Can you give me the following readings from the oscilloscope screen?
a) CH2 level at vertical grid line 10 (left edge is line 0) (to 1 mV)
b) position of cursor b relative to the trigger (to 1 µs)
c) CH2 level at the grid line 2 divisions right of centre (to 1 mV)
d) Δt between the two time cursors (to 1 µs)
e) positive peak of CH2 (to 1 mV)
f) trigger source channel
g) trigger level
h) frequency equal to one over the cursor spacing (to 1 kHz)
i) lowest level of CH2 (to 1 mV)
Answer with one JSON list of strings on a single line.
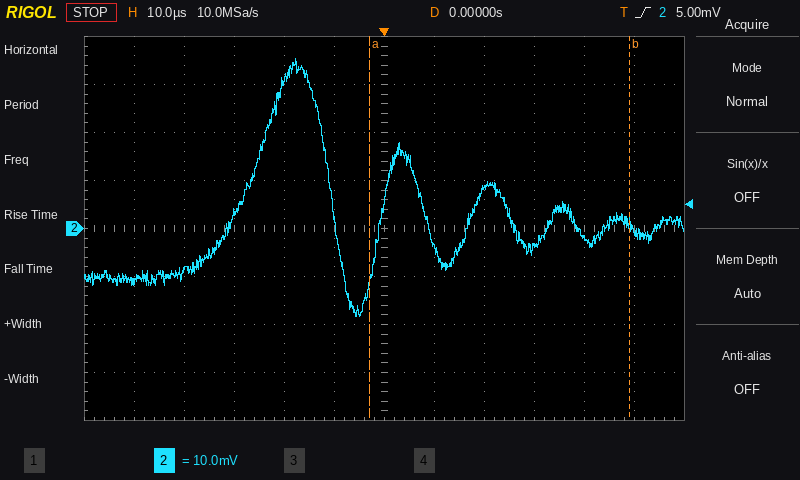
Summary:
["-2 mV", "+49 µs", "8 mV", "52 µs", "35 mV", "CH2", "5.00 mV", "19 kHz", "-18 mV"]
